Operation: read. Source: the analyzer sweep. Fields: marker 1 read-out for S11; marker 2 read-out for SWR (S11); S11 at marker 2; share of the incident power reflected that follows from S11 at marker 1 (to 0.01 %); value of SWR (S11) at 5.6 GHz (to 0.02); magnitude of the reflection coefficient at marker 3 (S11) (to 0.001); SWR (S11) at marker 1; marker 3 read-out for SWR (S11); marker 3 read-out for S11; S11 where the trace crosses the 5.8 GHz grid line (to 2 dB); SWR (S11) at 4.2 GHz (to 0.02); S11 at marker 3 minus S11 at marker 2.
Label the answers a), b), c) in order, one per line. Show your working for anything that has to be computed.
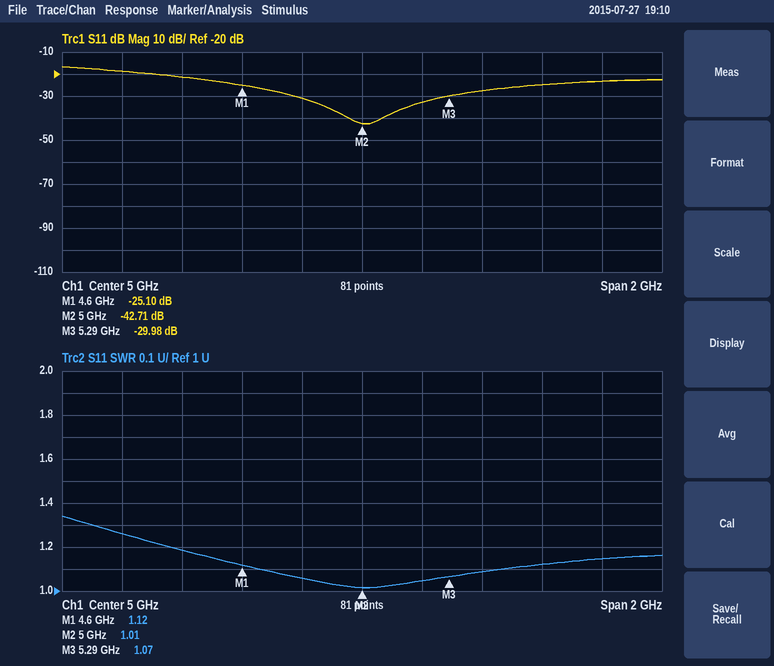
a) -25.10 dB
b) 1.01
c) -42.71 dB
d) 10^(-25.1/10) ≈ 0.31 %
e) 1.12
f) 10^(-29.98/20) ≈ 0.032
g) 1.12
h) 1.07
i) -29.98 dB
j) -24 dB
k) 1.26
l) -29.98 − (-42.71) = 12.73 dB
